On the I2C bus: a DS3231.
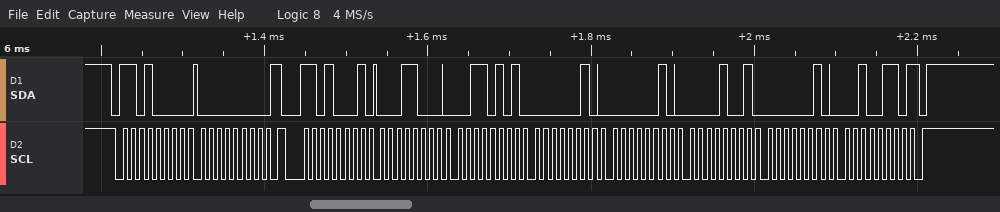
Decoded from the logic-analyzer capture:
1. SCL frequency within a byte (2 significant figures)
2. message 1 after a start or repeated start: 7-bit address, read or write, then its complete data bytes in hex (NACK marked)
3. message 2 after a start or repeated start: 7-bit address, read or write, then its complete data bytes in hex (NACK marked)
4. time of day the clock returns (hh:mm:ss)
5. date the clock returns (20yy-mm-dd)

100 kHz
0x68 write: 00
0x68 read: 18 35 02 02 09 02 26 NACK
02:35:18
2026-02-09
